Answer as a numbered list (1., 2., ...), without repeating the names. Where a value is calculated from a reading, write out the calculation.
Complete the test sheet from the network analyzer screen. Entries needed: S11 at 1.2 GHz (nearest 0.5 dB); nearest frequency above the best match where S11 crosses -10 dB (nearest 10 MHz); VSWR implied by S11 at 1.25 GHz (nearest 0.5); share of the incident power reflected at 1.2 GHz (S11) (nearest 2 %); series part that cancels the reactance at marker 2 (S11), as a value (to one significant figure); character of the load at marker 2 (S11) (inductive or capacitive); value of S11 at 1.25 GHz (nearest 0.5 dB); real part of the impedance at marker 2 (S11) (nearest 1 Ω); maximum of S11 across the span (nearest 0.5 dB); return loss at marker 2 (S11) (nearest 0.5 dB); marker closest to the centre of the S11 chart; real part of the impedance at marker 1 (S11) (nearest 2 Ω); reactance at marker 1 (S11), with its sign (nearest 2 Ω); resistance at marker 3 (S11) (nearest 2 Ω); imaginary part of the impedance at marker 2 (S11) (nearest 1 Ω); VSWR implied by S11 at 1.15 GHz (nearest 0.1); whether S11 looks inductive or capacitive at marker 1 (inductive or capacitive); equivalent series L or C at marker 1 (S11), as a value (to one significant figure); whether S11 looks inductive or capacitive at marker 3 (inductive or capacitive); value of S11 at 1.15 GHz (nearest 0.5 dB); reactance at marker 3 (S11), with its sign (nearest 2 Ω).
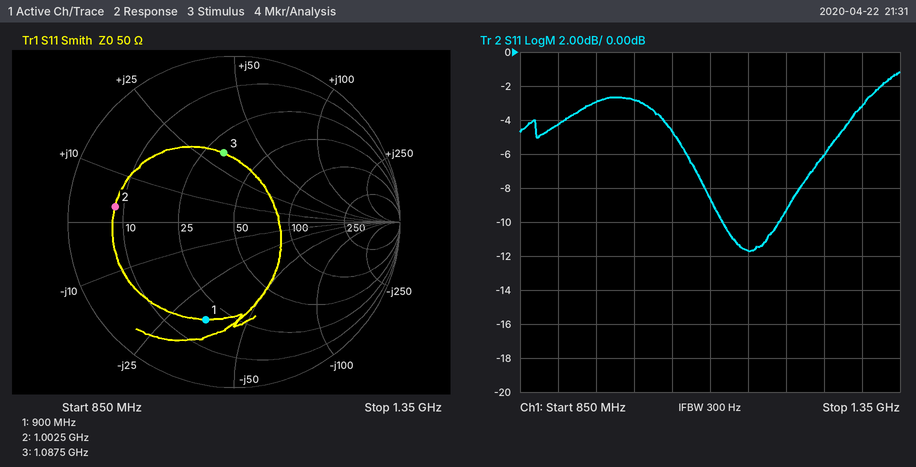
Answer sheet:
1. -9.5 dB
2. 1.19 GHz
3. |Γ| = 10^(-6/20) = 0.5012; VSWR = (1 + 0.5012)/(1 − 0.5012) ≈ 3.0
4. 10^(-9.5/10) ≈ 11.2 %, so 12 % to the nearest 2 %
5. C = 1/(2π × 1.0025 GHz × 3 Ω) ≈ 52.9 pF, so 50 pF to one significant figure
6. inductive
7. -6.0 dB
8. 8 Ω
9. -1.0 dB
10. 3.0 dB
11. marker 3
12. 18 Ω
13. -34 Ω
14. 32 Ω
15. +3 Ω
16. |Γ| = 10^(-11.5/20) = 0.2661; VSWR = (1 + 0.2661)/(1 − 0.2661) ≈ 1.7
17. capacitive
18. C = 1/(2π × 900 MHz × 34 Ω) ≈ 5 pF
19. inductive
20. -11.5 dB
21. +32 Ω
